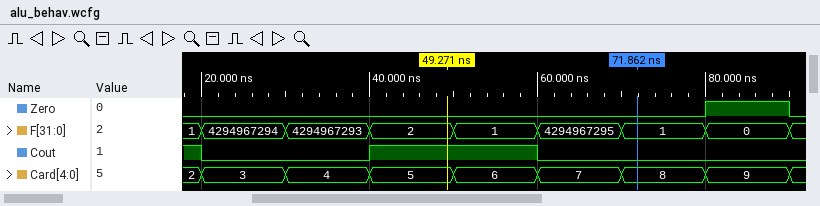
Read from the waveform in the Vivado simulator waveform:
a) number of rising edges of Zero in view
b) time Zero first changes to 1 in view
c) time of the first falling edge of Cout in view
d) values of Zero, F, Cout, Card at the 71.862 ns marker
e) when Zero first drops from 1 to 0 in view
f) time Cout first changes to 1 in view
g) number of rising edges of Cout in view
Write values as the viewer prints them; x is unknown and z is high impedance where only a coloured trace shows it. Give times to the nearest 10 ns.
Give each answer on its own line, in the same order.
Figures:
1
80 ns
20 ns
Zero=0, F=1, Cout=0, Card=8
90 ns
40 ns
1
